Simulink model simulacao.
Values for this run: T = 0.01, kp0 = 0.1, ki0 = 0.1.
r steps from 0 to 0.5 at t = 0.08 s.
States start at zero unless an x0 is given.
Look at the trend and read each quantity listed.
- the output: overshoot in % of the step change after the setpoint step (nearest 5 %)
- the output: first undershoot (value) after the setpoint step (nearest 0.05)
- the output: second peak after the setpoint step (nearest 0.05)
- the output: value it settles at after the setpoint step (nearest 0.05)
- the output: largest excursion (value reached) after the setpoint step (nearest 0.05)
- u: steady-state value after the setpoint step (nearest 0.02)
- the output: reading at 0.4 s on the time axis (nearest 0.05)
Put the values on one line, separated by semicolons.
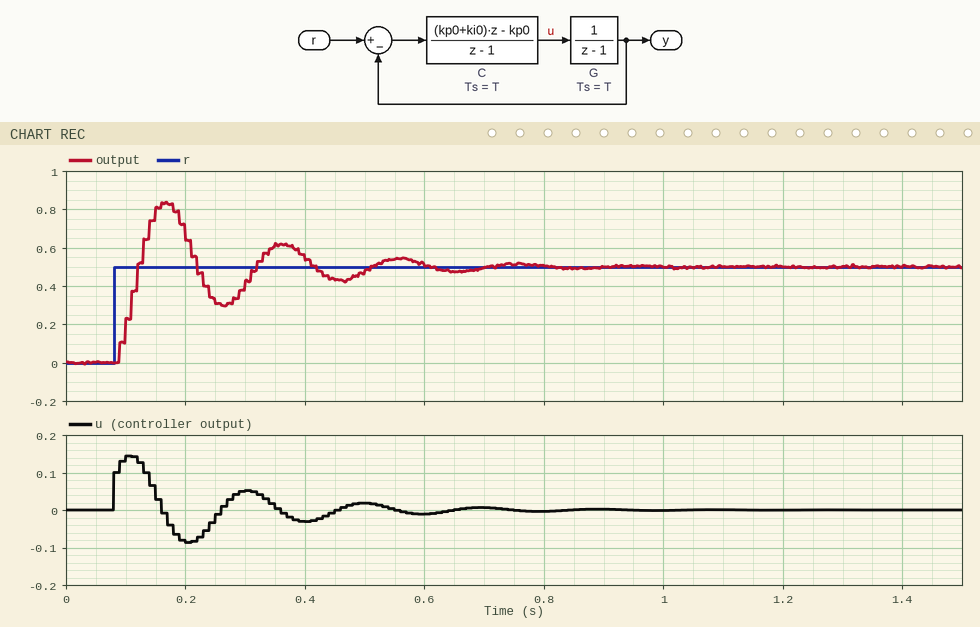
65 %; 0.30; 0.60; 0.50; 0.85; 0.00; 0.55
